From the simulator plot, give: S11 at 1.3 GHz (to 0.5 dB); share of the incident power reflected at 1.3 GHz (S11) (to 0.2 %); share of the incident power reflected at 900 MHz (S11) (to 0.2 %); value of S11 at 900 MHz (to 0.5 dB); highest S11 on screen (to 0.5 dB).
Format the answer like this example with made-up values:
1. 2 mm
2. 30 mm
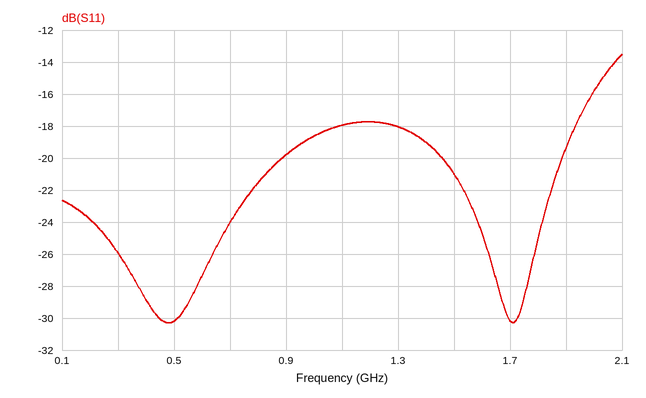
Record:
1. -18.0 dB
2. 1.6 %
3. 1.0 %
4. -20.0 dB
5. -13.5 dB
